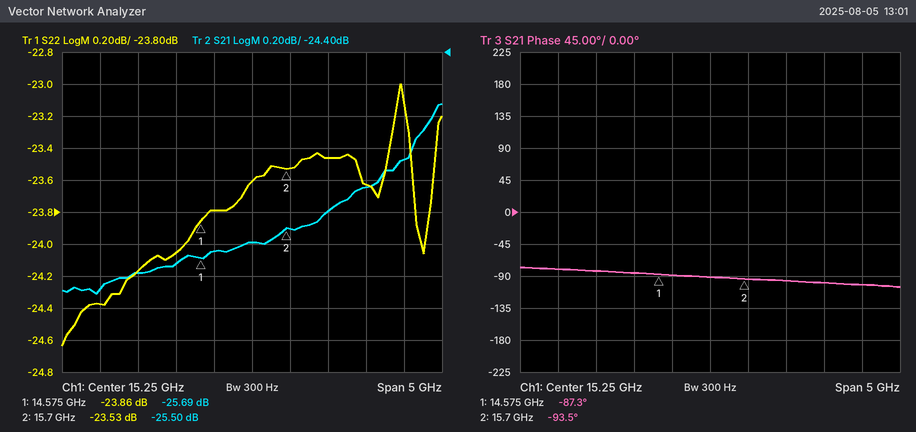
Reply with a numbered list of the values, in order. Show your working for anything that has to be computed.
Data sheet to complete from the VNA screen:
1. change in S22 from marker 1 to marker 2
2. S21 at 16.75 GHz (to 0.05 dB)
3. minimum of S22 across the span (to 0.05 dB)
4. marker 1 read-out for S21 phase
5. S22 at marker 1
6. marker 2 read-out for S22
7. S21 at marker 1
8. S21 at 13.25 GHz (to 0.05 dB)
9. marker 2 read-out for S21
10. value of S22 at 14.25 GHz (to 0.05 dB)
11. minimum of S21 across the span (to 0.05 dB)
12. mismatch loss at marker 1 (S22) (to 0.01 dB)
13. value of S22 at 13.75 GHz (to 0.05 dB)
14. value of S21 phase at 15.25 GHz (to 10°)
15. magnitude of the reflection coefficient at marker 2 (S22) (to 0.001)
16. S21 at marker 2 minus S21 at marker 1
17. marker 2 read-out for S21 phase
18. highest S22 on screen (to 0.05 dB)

1. -23.53 − (-23.86) = 0.33 dB
2. -25.25 dB
3. -24.65 dB
4. -87.3°
5. -23.86 dB
6. -23.53 dB
7. -25.69 dB
8. -25.90 dB
9. -25.50 dB
10. -24.05 dB
11. -25.90 dB
12. −10 log10(1 − 10^(-23.86/10)) ≈ 0.02 dB
13. -24.15 dB
14. -90°
15. 10^(-23.53/20) ≈ 0.067
16. -25.5 − (-25.69) = 0.19 dB
17. -93.5°
18. -23.00 dB
